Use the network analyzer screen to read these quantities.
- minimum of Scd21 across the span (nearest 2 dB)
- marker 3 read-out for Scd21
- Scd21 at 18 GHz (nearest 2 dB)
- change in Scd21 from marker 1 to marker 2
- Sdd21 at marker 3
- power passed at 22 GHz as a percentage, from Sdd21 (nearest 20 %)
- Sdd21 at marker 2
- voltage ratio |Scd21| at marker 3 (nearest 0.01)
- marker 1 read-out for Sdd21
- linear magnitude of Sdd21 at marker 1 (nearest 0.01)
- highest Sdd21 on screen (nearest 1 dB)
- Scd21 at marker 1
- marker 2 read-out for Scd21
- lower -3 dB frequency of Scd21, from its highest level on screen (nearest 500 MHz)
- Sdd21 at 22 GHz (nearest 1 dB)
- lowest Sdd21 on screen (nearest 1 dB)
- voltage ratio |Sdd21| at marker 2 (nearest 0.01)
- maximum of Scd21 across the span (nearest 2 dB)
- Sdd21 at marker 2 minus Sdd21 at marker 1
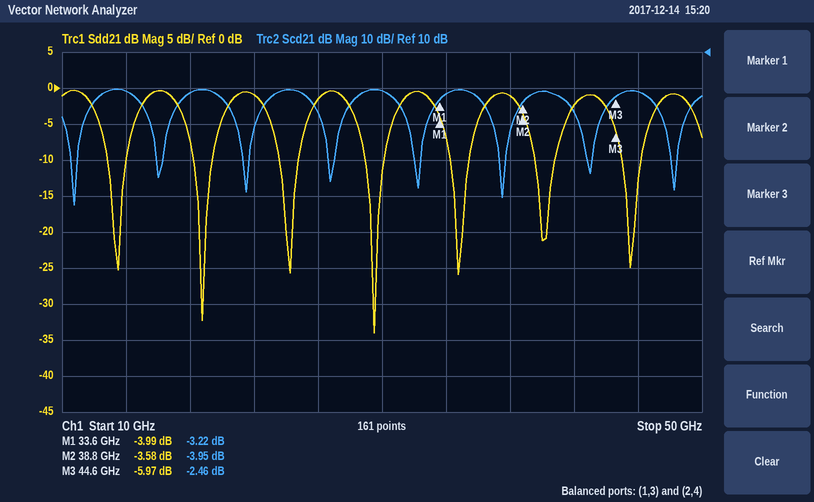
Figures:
-32 dB
-2.46 dB
-2 dB
-0.73 dB
-5.97 dB
80 %
-3.58 dB
0.75
-3.99 dB
0.63
0 dB
-3.22 dB
-3.95 dB
12.0 GHz
-1 dB
-34 dB
0.66
0 dB
0.41 dB
